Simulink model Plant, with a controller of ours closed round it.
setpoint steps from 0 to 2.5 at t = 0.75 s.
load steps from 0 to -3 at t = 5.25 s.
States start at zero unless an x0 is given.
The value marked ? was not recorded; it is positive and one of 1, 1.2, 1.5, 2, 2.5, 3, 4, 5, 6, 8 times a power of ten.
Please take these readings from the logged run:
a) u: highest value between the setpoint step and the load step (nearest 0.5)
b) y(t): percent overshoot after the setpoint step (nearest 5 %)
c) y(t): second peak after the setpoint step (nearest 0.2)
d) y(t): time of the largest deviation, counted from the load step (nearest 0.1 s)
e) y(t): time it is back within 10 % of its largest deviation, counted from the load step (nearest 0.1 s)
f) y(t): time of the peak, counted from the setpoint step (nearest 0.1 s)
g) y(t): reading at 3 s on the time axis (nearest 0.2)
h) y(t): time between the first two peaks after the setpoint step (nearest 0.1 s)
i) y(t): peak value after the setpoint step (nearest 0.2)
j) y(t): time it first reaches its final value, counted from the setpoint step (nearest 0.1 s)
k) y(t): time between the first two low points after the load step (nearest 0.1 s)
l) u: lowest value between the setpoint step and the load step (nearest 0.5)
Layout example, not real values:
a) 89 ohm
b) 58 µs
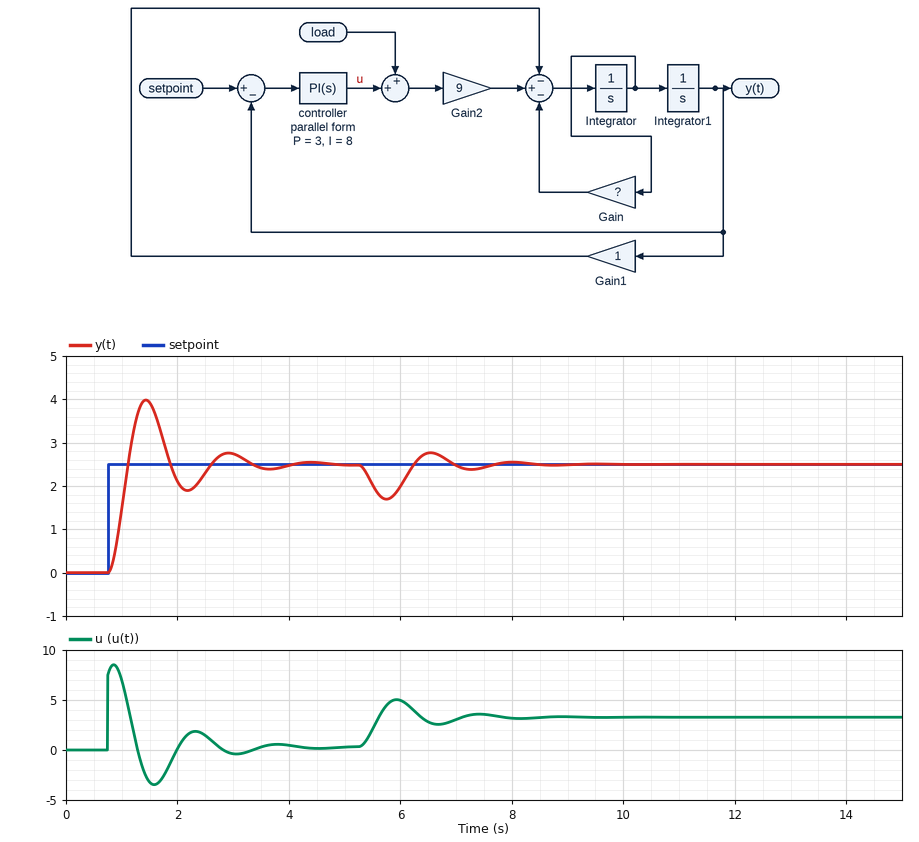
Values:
a) 8.5
b) 60 %
c) 2.8
d) 0.5 s
e) 2.2 s
f) 0.7 s
g) 2.8
h) 1.5 s
i) 4.0
j) 0.4 s
k) 1.5 s
l) -3.5
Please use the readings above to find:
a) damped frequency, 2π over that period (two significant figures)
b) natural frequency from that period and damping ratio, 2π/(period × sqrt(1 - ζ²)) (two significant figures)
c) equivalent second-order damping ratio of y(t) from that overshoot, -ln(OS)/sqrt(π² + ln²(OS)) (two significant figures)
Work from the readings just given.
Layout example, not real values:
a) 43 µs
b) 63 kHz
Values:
a) 4.2 rad/s
b) 4.2 rad/s
c) 0.16
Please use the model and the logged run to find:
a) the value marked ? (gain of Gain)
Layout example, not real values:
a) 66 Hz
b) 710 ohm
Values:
a) 6
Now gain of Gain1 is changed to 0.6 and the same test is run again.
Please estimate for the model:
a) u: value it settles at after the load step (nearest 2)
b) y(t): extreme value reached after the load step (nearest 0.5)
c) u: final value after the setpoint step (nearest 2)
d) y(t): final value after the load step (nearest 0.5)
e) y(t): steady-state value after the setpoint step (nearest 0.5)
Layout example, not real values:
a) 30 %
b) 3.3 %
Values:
a) 4
b) 1.5
c) 0
d) 2.5
e) 2.5
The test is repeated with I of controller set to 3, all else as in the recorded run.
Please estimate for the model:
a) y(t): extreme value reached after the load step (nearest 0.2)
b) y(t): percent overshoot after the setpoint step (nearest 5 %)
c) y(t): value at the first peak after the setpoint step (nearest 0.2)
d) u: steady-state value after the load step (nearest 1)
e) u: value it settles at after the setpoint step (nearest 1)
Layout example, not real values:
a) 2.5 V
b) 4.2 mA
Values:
a) 1.6
b) 30 %
c) 3.2
d) 3
e) 0
